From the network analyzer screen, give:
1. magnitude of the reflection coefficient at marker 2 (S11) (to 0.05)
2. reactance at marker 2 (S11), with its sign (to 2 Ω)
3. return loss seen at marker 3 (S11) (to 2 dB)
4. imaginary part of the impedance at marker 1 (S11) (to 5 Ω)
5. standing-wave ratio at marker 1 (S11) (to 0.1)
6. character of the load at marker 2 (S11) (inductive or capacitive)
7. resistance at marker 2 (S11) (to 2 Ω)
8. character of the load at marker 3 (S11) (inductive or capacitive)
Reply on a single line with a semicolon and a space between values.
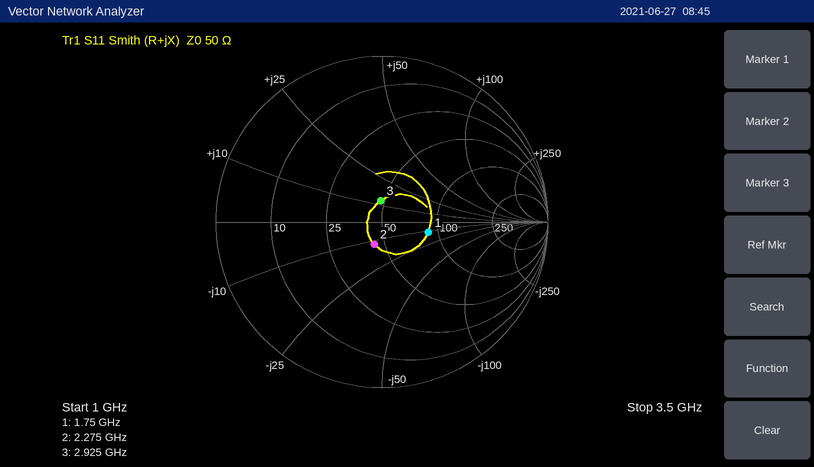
0.15; -12 Ω; 18 dB; -10 Ω; 1.8; capacitive; 44 Ω; inductive
